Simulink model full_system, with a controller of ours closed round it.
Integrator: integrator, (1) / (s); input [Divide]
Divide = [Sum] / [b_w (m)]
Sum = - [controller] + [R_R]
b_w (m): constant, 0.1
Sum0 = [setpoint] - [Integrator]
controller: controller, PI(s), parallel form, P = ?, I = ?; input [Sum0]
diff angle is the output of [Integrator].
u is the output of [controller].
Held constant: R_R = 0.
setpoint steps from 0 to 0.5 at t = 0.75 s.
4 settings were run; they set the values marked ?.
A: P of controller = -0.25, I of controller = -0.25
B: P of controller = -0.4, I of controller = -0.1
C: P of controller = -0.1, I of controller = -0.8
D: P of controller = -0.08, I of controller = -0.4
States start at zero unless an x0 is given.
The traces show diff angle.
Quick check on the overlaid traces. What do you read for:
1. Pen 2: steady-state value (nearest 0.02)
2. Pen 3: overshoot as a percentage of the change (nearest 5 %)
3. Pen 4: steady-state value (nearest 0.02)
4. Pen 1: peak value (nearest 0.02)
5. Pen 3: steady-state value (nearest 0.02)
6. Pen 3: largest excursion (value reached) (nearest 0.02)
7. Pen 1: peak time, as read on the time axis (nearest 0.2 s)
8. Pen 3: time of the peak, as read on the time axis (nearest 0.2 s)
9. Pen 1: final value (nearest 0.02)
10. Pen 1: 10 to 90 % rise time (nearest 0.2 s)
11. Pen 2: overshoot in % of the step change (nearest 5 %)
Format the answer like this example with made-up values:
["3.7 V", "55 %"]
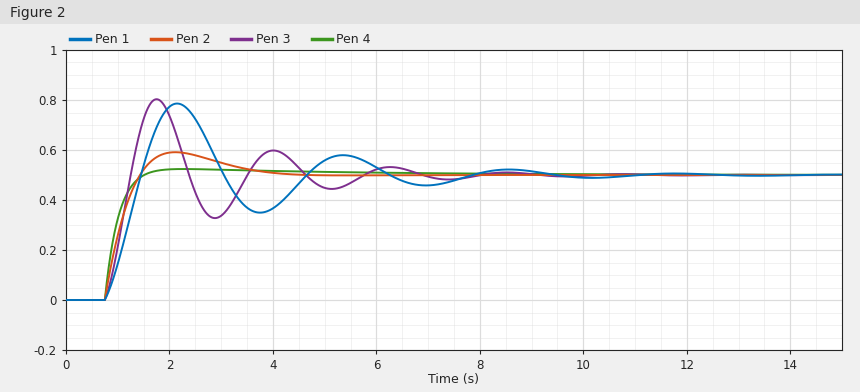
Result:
["0.50", "60 %", "0.50", "0.78", "0.50", "0.80", "2.2 s", "1.8 s", "0.50", "0.6 s", "20 %"]
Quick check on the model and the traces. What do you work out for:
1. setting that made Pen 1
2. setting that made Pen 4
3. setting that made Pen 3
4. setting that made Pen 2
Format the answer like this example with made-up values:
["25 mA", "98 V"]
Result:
["D", "B", "C", "A"]
